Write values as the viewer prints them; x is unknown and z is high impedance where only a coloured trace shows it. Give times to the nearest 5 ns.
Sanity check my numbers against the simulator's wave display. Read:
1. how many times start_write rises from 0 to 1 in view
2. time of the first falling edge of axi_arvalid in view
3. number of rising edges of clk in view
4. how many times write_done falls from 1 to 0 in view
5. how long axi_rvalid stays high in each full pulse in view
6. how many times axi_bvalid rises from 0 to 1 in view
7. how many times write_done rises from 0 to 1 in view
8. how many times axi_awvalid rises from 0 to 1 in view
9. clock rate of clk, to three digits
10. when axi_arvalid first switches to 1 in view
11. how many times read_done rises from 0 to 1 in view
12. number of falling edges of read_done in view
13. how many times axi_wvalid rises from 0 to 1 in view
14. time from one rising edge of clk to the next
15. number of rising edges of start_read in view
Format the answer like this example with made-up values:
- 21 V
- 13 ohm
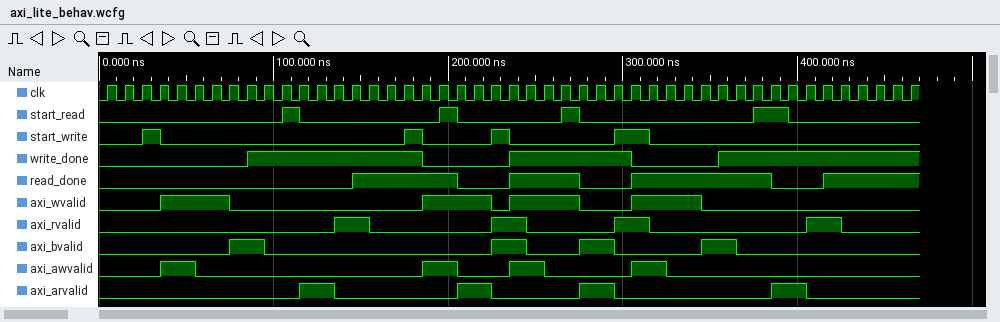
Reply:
- 4
- 135 ns
- 47
- 2
- 20 ns, 20 ns, 20 ns, 20 ns
- 4
- 3
- 4
- 100 MHz
- 115 ns
- 4
- 3
- 4
- 10 ns
- 4
